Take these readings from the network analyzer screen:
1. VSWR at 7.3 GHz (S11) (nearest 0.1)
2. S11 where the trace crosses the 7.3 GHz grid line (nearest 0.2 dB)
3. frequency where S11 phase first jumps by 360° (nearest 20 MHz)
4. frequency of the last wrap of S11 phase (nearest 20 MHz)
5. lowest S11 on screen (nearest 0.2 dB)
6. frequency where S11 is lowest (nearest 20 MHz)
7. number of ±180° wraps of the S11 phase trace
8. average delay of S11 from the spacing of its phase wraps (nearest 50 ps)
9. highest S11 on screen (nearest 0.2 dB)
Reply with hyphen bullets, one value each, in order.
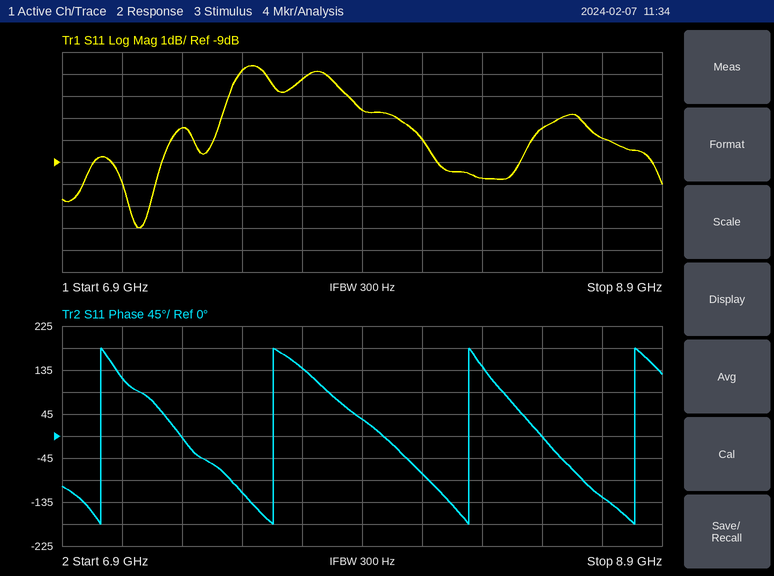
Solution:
- 2.5
- -7.4 dB
- 7.02 GHz
- 8.80 GHz
- -12.0 dB
- 7.16 GHz
- 4
- 1.70 ns
- -4.6 dB
